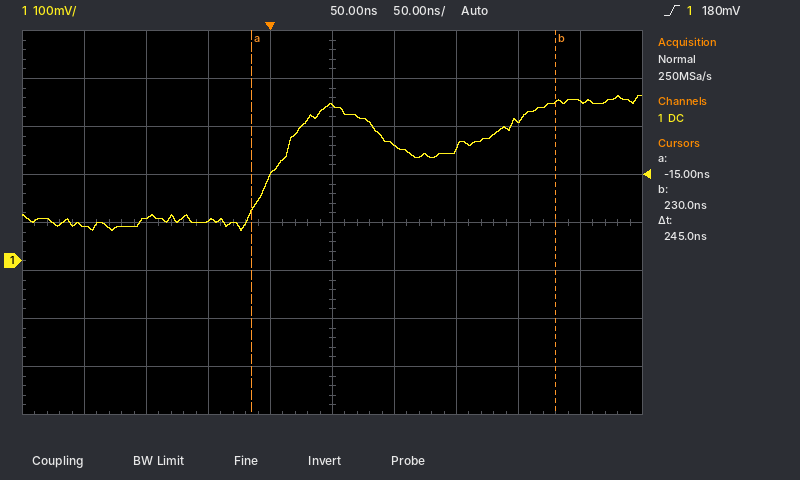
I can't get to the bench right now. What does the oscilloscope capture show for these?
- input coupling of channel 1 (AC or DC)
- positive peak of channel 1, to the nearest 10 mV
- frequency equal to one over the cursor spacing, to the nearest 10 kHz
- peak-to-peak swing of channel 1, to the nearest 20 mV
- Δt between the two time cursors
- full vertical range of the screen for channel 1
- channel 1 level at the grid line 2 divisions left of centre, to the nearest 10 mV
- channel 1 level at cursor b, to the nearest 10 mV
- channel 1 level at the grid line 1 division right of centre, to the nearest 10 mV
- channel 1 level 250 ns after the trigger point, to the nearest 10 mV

DC
340 mV
4.08 MHz
280 mV
245 ns
800 mV
80 mV
330 mV
240 mV
330 mV
